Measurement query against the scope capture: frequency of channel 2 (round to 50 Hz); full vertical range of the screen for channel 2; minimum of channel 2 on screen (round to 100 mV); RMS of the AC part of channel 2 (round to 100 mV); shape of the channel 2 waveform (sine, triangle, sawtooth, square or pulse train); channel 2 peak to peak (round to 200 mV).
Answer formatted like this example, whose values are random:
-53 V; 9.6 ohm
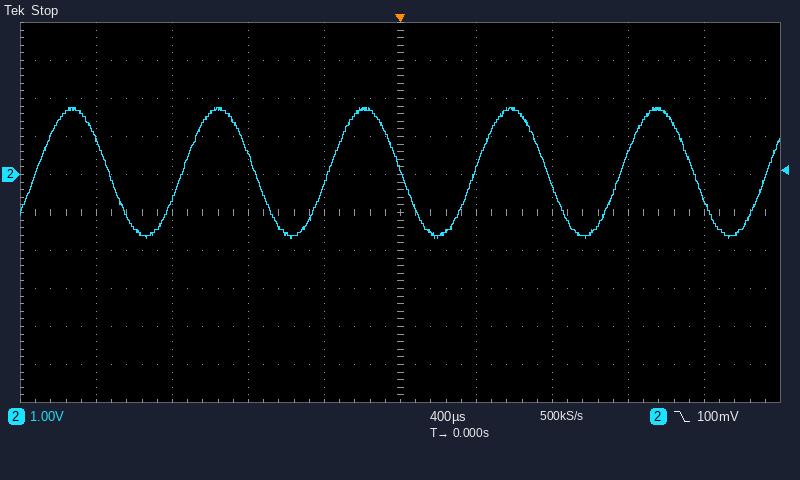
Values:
1.30 kHz; 10 V; -1.7 V; 1.2 V; sine; 3.4 V
